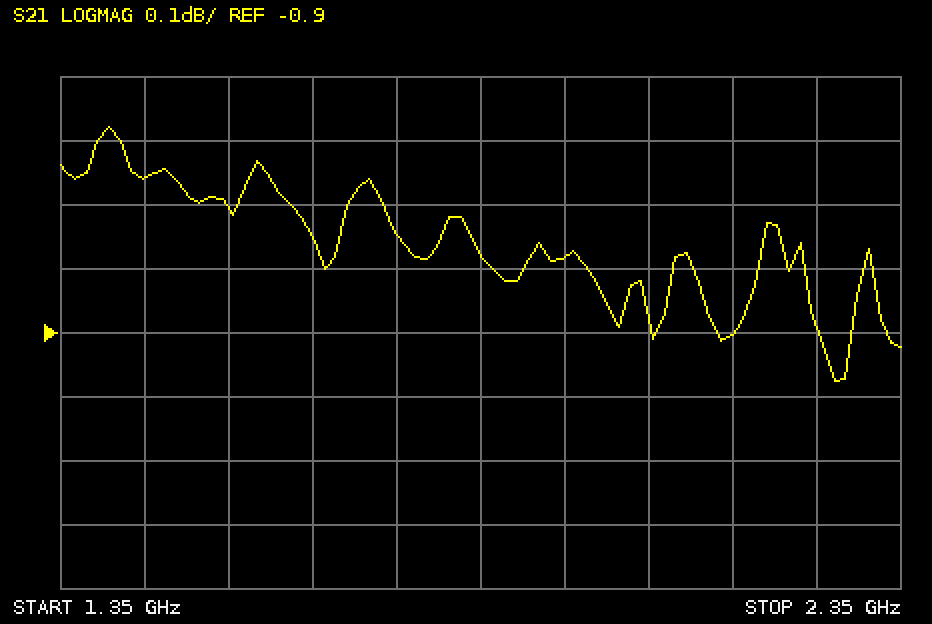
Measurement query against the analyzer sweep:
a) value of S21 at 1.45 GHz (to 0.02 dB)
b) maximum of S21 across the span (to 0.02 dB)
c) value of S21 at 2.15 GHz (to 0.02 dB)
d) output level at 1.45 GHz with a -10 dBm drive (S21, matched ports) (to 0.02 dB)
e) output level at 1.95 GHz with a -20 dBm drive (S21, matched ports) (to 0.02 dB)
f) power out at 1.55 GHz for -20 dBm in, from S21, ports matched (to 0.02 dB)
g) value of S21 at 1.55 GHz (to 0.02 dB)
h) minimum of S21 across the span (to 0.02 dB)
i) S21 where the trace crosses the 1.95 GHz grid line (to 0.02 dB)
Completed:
-0.66 dB
-0.58 dB
-0.90 dB
-10.66 dBm
-20.78 dBm
-20.70 dBm
-0.70 dB
-0.98 dB
-0.78 dB
